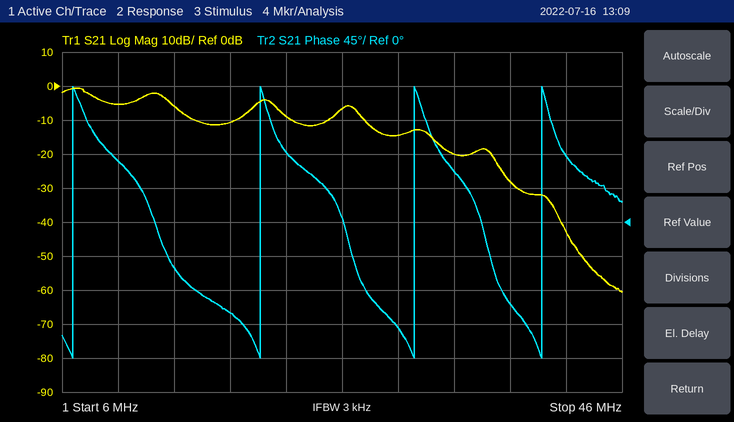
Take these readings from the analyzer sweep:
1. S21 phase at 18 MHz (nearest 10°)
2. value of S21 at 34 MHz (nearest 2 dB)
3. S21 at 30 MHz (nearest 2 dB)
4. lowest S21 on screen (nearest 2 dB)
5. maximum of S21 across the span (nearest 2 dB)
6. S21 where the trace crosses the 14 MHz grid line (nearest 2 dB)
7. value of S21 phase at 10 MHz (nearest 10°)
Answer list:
-120°
-20 dB
-14 dB
-60 dB
0 dB
-6 dB
80°
